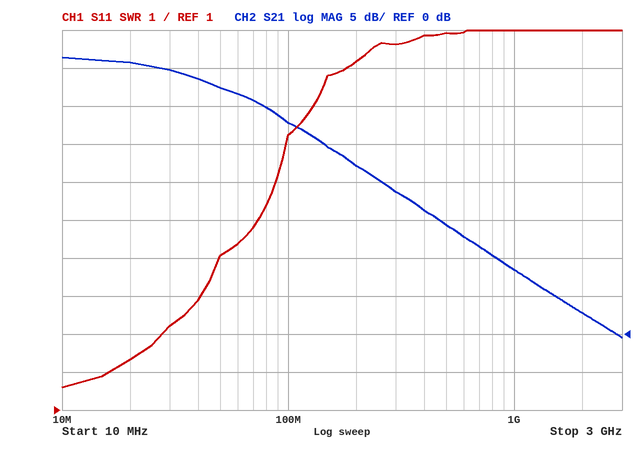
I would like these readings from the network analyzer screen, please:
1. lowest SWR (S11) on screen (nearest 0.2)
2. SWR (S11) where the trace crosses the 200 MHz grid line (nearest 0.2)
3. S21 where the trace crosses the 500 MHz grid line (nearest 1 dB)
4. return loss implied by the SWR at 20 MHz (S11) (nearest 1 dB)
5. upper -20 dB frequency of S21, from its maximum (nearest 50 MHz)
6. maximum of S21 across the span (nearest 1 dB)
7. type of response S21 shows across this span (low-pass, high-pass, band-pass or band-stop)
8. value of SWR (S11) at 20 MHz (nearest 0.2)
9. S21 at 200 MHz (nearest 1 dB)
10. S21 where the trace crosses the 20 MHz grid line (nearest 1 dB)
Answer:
1.6
10.2
14 dB
8 dB
400 MHz
36 dB
low-pass
2.4
22 dB
36 dB
